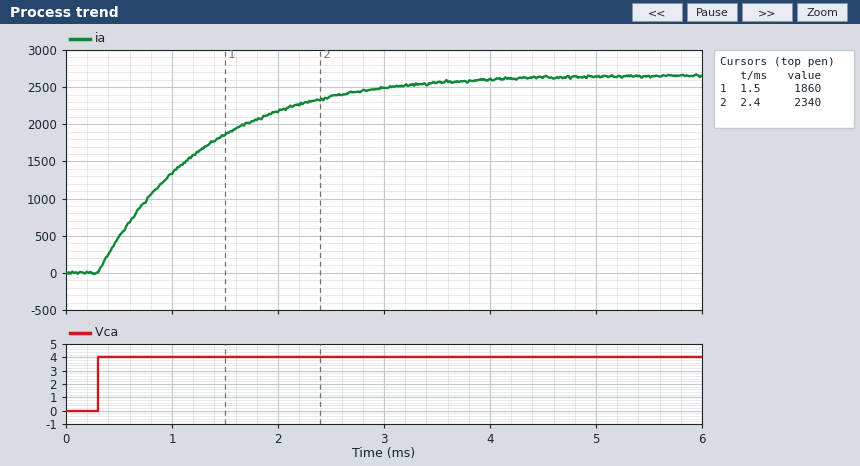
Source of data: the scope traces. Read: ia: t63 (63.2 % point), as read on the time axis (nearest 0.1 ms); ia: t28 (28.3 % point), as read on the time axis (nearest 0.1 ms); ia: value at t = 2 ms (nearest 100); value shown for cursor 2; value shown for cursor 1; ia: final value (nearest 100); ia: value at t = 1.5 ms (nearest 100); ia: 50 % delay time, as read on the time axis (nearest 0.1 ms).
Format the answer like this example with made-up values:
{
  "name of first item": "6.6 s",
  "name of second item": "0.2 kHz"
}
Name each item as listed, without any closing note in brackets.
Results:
{
  "ia: t63 (63.2 % point), as read on the time axis": "1.3 ms",
  "ia: t28 (28.3 % point), as read on the time axis": "0.6 ms",
  "ia: value at t = 2 ms": "2200",
  "value shown for cursor 2": "2340",
  "value shown for cursor 1": "1860",
  "ia: final value": "2700",
  "ia: value at t = 1.5 ms": "1900",
  "ia: 50 % delay time, as read on the time axis": "1.0 ms"
}
